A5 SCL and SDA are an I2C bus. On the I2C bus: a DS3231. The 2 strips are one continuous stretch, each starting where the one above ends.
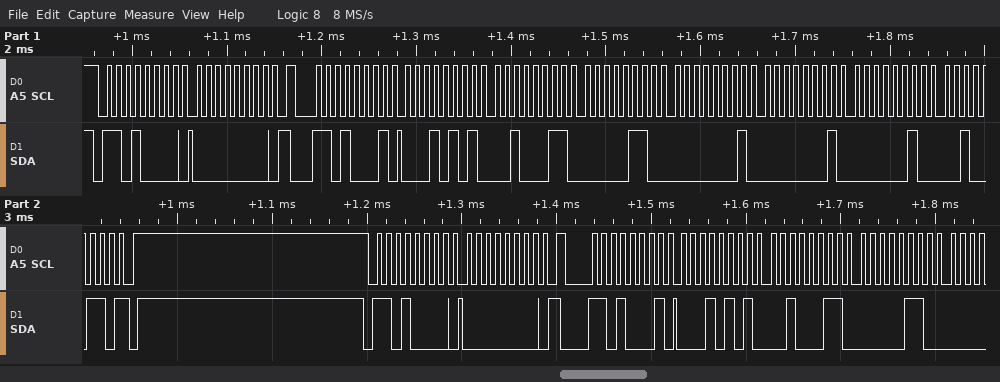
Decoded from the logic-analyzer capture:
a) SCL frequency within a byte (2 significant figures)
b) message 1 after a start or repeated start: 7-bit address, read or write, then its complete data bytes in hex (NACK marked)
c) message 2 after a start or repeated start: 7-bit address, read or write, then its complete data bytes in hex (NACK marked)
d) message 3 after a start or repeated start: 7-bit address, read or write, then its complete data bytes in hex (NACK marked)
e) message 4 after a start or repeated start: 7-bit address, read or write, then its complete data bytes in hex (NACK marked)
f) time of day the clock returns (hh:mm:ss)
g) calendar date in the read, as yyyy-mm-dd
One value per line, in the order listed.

100 kHz
0x68 write: 00
0x68 read: 15 23 06 01 01 02 26 NACK
0x68 write: 00
0x68 read: 15 23 06
06:23:15
2026-02-01
